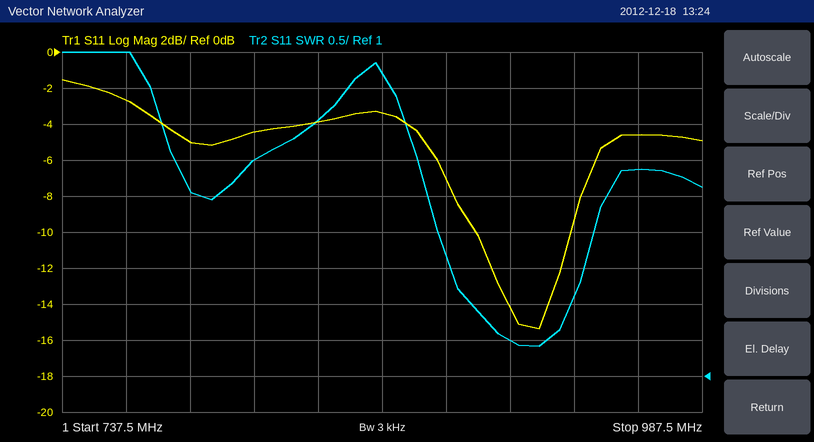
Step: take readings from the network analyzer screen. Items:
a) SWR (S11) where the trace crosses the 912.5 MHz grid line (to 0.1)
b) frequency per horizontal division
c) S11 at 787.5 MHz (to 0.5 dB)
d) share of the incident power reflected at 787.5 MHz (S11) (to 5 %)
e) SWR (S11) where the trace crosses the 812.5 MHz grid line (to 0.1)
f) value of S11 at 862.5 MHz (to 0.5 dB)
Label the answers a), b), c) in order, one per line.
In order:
a) 1.5
b) 25 MHz
c) -5.0 dB
d) 30 %
e) 4.0
f) -3.5 dB
